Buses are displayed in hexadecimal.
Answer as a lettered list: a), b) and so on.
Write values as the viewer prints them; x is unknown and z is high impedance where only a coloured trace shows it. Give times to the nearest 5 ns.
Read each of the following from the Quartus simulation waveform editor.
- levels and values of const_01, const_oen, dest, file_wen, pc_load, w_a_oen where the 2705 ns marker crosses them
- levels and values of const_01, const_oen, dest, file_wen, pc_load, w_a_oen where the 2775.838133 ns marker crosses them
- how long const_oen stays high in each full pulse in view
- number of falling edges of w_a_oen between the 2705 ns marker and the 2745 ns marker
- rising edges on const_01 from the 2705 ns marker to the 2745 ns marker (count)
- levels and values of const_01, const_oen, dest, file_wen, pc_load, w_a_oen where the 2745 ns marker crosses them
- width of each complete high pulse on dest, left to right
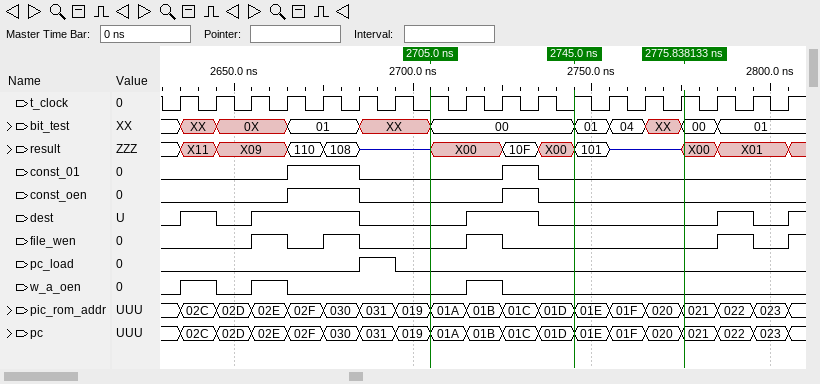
a) const_01=0, const_oen=0, dest=0, file_wen=0, pc_load=0, w_a_oen=0
b) const_01=0, const_oen=0, dest=0, file_wen=0, pc_load=0, w_a_oen=0
c) 20 ns, 10 ns
d) 1
e) 1
f) const_01=0, const_oen=0, dest=0, file_wen=0, pc_load=0, w_a_oen=0
g) 10 ns, 30 ns, 20 ns, 10 ns
